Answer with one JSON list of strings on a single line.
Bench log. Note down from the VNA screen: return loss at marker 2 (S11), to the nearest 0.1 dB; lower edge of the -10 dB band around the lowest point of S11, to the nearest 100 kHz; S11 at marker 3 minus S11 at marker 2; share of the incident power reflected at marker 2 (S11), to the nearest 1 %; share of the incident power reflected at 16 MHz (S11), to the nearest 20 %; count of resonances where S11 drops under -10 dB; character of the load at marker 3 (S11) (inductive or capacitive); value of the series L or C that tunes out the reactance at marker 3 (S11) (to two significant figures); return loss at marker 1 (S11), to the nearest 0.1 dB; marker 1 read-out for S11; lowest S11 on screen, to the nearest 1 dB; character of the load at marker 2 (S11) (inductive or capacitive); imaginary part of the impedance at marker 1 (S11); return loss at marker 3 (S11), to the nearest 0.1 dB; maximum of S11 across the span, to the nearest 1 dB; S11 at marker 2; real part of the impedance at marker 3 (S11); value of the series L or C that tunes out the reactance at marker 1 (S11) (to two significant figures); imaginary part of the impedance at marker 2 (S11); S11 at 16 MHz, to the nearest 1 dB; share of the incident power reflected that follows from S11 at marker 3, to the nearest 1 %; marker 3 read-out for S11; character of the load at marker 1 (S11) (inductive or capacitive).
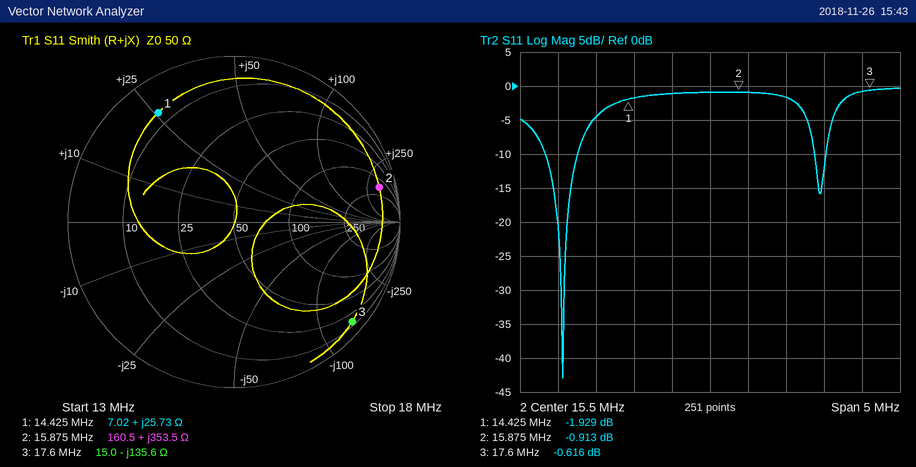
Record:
["0.9 dB", "13.3 MHz", "0.297 dB", "81 %", "80 %", "2", "capacitive", "1.2 µH", "1.9 dB", "-1.929 dB", "-43 dB", "inductive", "+25.73 Ω", "0.6 dB", "0 dB", "-0.913 dB", "15.0 Ω", "430 pF", "+353.5 Ω", "-1 dB", "87 %", "-0.616 dB", "inductive"]
